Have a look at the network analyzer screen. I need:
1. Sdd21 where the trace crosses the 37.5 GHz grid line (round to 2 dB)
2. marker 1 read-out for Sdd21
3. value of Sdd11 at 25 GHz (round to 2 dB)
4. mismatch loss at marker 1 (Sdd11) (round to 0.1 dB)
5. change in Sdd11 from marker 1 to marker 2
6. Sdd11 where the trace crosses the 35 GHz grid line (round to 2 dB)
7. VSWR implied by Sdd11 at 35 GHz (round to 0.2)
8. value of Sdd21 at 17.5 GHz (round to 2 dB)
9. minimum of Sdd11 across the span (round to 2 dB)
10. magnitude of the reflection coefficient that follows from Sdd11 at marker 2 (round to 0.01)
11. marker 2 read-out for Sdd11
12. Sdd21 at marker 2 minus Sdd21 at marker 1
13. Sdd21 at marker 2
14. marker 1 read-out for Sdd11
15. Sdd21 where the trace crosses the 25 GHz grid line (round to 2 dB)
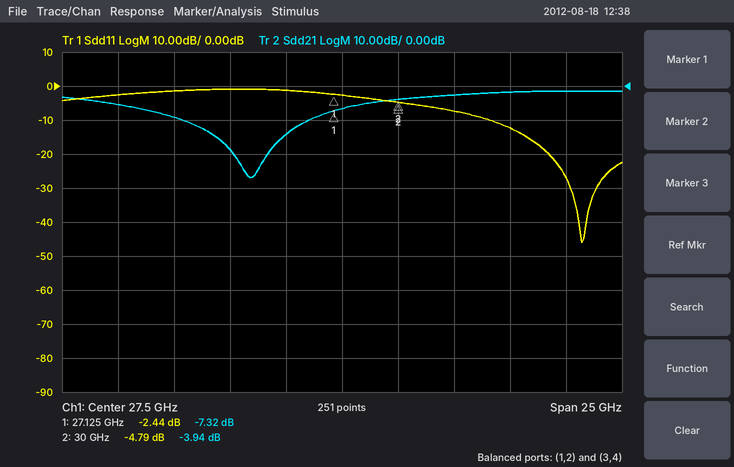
-2 dB
-7.32 dB
-2 dB
3.7 dB
-2.35 dB
-12 dB
1.6
-6 dB
-46 dB
0.58
-4.79 dB
3.38 dB
-3.94 dB
-2.44 dB
-14 dB
